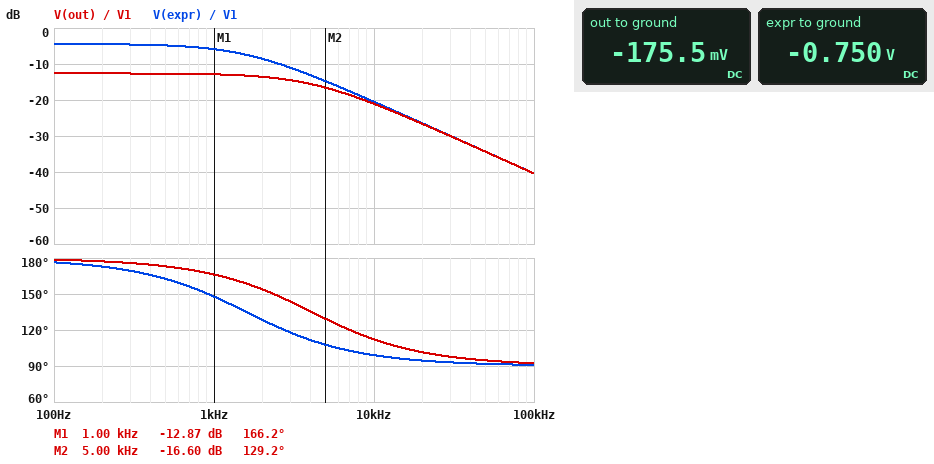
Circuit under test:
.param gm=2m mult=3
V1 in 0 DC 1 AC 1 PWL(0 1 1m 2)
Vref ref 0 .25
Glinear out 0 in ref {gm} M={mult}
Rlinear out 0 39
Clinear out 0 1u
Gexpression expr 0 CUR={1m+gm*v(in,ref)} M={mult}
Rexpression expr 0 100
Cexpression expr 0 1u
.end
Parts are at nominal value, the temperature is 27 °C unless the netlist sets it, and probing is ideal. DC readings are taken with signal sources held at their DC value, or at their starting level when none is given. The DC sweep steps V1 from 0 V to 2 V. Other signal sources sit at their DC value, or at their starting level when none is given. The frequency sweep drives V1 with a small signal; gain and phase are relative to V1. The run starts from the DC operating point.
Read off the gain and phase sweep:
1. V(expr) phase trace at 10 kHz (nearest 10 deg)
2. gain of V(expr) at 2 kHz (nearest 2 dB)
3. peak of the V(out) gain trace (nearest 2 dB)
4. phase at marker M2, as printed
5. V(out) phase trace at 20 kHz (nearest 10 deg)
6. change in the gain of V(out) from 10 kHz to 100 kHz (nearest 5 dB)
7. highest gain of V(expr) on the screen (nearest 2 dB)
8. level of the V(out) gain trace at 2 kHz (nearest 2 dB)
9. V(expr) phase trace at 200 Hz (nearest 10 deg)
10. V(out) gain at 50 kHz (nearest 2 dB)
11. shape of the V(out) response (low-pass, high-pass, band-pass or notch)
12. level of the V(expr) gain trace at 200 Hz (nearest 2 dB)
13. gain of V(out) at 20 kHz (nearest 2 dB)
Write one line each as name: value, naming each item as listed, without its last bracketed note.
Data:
V(expr) phase trace at 10 kHz: 100 deg
gain of V(expr) at 2 kHz: -8 dB
peak of the V(out) gain trace: -12 dB
phase at marker M2, as printed: 129.2 deg
V(out) phase trace at 20 kHz: 100 deg
change in the gain of V(out) from 10 kHz to 100 kHz: -20 dB
highest gain of V(expr) on the screen: -4 dB
level of the V(out) gain trace at 2 kHz: -14 dB
V(expr) phase trace at 200 Hz: 170 deg
V(out) gain at 50 kHz: -34 dB
shape of the V(out) response: low-pass
level of the V(expr) gain trace at 200 Hz: -4 dB
gain of V(out) at 20 kHz: -26 dB
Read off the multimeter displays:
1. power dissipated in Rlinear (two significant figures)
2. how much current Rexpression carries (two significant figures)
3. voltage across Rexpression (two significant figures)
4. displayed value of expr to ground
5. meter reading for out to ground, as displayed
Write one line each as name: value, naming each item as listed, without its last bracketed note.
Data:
power dissipated in Rlinear: 790 µW
how much current Rexpression carries: 7.5 mA
voltage across Rexpression: 750 mV
displayed value of expr to ground: -0.750 V
meter reading for out to ground, as displayed: -175.5 mV
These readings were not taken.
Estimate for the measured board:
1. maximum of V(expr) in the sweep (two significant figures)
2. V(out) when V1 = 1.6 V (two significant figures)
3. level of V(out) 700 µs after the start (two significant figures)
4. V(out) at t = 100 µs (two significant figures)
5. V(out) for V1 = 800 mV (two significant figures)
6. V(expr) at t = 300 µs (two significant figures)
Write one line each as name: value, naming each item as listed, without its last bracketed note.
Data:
maximum of V(expr) in the sweep: -150 mV
V(out) when V1 = 1.6 V: -320 mV
level of V(out) 700 µs after the start: -330 mV
V(out) at t = 100 µs: -190 mV
V(out) for V1 = 800 mV: -130 mV
V(expr) at t = 300 µs: -870 mV
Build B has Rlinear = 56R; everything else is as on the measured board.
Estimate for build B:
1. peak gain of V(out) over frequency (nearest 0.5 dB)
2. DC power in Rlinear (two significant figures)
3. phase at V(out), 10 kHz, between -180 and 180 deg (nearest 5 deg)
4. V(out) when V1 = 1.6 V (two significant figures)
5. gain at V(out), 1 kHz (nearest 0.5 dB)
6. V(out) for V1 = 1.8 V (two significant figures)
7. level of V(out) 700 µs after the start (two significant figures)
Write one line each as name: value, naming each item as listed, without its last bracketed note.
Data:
peak gain of V(out) over frequency: -9.5 dB
DC power in Rlinear: 1.1 mW
phase at V(out), 10 kHz, between -180 and 180 deg: 105 deg
V(out) when V1 = 1.6 V: -450 mV
gain at V(out), 1 kHz: -10.0 dB
V(out) for V1 = 1.8 V: -520 mV
level of V(out) 700 µs after the start: -470 mV
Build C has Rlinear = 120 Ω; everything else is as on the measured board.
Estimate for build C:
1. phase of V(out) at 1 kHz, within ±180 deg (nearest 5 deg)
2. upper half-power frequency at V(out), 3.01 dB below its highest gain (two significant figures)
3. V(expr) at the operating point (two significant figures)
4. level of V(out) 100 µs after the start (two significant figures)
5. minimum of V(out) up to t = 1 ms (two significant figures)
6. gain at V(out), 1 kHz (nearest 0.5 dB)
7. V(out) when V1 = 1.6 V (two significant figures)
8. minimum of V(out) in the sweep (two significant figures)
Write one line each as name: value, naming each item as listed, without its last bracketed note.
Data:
phase of V(out) at 1 kHz, within ±180 deg: 145 deg
upper half-power frequency at V(out), 3.01 dB below its highest gain: 1.3 kHz
V(expr) at the operating point: -750 mV
level of V(out) 100 µs after the start: -560 mV
minimum of V(out) up to t = 1 ms: -1.2 V
gain at V(out), 1 kHz: -5.0 dB
V(out) when V1 = 1.6 V: -970 mV
minimum of V(out) in the sweep: -1.3 V
